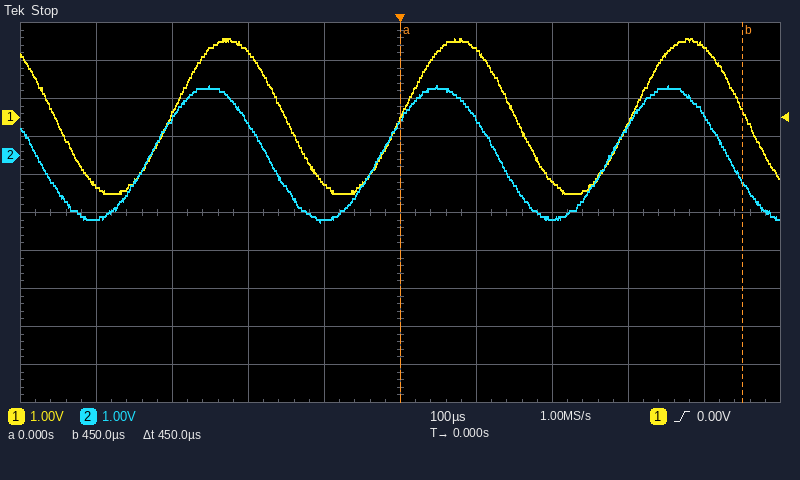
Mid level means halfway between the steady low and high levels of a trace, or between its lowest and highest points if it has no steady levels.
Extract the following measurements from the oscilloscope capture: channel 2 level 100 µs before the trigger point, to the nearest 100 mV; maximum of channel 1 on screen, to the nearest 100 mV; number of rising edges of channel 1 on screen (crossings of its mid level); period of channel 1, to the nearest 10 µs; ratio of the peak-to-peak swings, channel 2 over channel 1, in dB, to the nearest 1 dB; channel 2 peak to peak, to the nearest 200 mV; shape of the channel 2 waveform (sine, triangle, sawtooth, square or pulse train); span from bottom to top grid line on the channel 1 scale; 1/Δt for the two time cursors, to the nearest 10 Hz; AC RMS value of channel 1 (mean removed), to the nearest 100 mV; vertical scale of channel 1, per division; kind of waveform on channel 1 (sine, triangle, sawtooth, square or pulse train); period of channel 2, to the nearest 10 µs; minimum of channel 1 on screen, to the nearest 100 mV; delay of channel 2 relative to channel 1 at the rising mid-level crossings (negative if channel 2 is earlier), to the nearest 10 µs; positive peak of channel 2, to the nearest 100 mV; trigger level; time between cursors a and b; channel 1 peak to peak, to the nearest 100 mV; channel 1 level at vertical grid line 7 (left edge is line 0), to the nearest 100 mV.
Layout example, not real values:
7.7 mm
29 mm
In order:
-1.7 V
2.1 V
3
300 µs
-1 dB
3.6 V
sine
10 V
2.22 kHz
1.4 V
1 V
sine
300 µs
-2.0 V
-30 µs
1.8 V
0.00 V
450 µs
4.1 V
-1.7 V
